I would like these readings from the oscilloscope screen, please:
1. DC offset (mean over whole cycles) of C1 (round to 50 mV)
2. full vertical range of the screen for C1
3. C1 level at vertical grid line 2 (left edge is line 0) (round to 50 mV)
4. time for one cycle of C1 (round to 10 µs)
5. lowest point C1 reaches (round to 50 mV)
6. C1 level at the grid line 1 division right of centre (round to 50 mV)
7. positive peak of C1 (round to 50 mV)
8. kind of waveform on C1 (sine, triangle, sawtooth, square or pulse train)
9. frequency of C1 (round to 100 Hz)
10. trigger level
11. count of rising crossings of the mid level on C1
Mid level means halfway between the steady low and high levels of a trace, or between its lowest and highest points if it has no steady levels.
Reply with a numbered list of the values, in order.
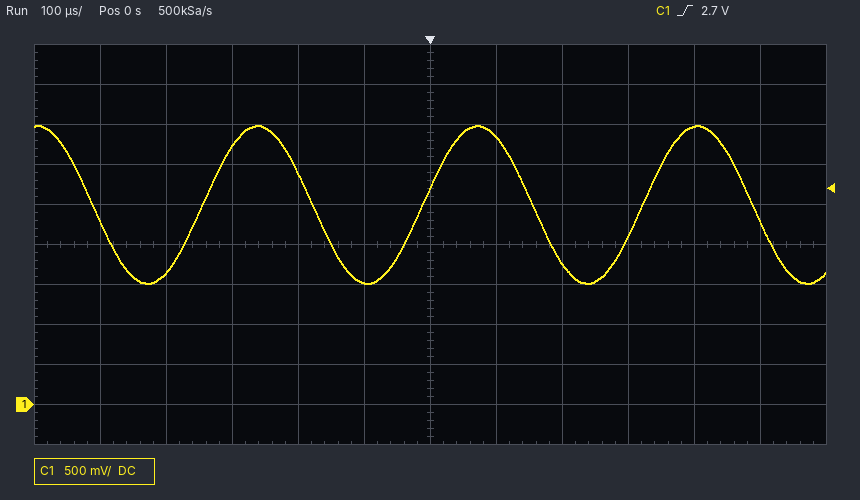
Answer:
1. 2.50 V
2. 5 V
3. 1.65 V
4. 330 µs
5. 1.50 V
6. 3.35 V
7. 3.50 V
8. sine
9. 3.0 kHz
10. 2.7 V
11. 3
